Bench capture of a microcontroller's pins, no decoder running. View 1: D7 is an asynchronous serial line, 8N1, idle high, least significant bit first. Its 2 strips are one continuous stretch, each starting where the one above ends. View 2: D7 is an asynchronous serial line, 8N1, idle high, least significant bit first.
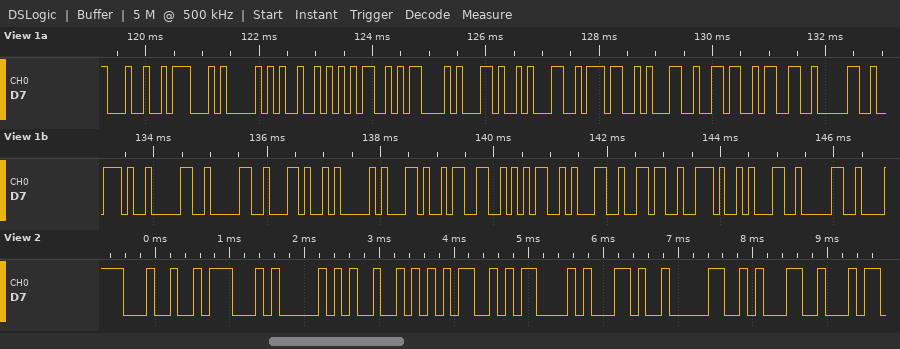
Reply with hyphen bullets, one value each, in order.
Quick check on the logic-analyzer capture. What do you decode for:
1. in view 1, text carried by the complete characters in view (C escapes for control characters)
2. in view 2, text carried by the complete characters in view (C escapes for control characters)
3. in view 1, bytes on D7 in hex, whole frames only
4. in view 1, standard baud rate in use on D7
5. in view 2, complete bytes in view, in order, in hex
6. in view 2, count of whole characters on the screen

- "$GPRMC,171630.00,A,3516.10"
- "$GPRMC,01"
- 24 47 50 52 4D 43 2C 31 37 31 36 33 30 2E 30 30 2C 41 2C 33 35 31 36 2E 31 30
- 9600 baud
- 0x24 0x47 0x50 0x52 0x4D 0x43 0x2C 0x30 0x31
- 9
